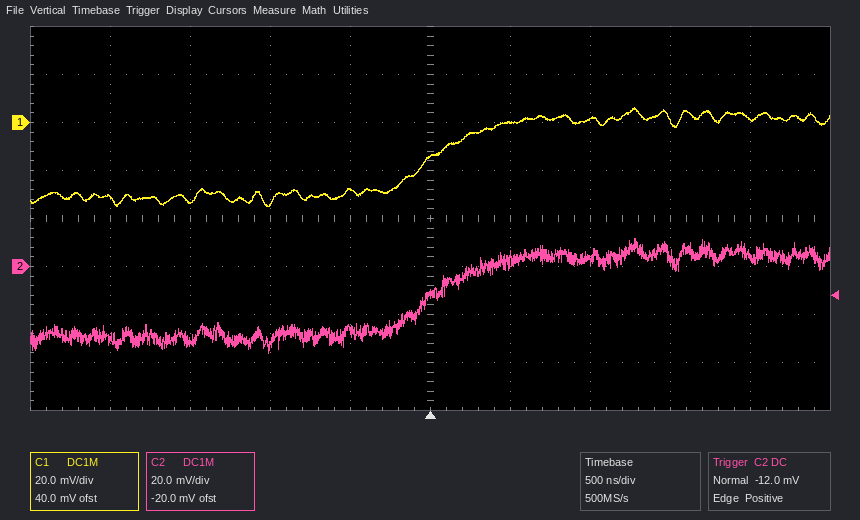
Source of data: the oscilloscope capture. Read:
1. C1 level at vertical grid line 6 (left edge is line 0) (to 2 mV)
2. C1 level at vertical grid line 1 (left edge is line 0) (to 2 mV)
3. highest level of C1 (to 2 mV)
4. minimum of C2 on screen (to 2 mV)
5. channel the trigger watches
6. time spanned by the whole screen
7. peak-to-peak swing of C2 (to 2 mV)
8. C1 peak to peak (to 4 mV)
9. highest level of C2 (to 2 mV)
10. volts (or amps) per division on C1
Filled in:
0 mV
-32 mV
6 mV
-36 mV
C2
5 µs
48 mV
40 mV
12 mV
20 mV
